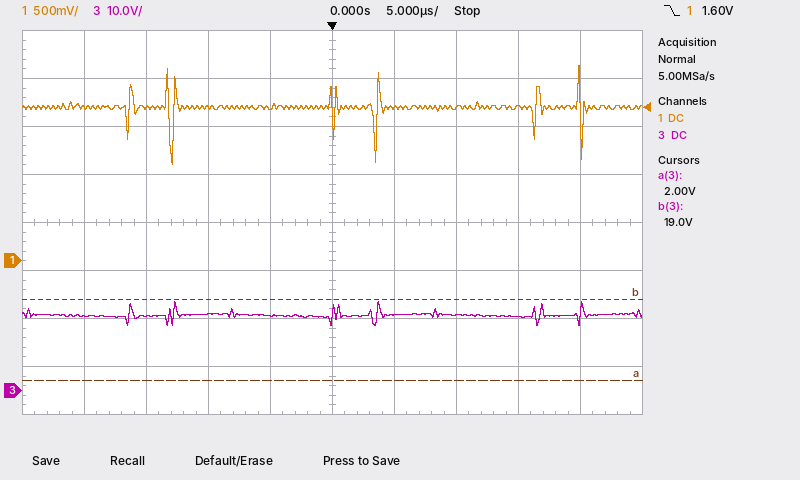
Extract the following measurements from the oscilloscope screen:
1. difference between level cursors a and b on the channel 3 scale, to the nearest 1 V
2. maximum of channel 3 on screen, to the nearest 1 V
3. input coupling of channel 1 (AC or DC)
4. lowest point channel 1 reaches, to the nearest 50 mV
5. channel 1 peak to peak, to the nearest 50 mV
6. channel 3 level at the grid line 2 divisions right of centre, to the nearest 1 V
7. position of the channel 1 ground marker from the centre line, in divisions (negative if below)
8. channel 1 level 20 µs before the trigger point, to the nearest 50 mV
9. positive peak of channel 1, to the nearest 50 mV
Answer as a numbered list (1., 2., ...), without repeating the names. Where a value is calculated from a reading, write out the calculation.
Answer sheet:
1. 17 V
2. 19 V
3. DC
4. 1.00 V
5. 2.05 V − (1.00 V) = 1.05 V
6. 16 V
7. -0.8 div
8. 1.60 V
9. 2.05 V
